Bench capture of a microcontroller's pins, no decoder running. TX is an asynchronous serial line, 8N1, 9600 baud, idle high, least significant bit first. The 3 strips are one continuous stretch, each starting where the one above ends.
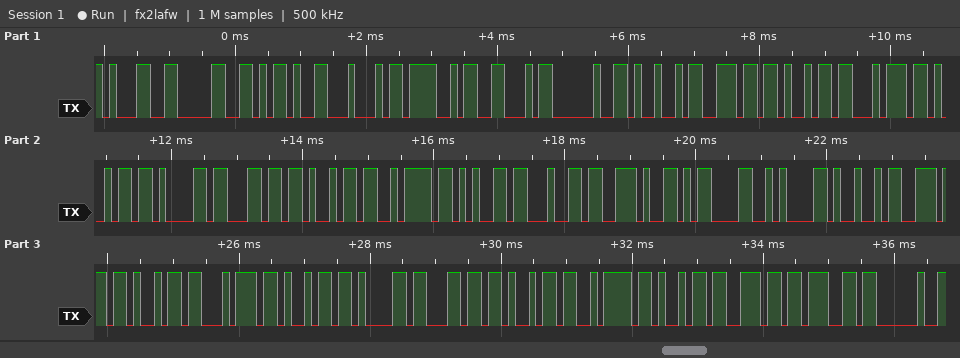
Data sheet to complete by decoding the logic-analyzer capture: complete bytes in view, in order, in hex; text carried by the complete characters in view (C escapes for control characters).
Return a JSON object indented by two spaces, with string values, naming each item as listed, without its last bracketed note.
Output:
{
  "complete bytes in view, in order, in hex": "31 30 2D 44 4F 46 20 49 6E 69 74 69 61 6C 69 7A 65 64 2E 0D 0A 49 6E 69 74 69 61 6C 69 7A 69 6E 67 20",
  "text carried by the complete characters in view": "\"10-DOF Initialized.\\r\\nInitializing \""
}
